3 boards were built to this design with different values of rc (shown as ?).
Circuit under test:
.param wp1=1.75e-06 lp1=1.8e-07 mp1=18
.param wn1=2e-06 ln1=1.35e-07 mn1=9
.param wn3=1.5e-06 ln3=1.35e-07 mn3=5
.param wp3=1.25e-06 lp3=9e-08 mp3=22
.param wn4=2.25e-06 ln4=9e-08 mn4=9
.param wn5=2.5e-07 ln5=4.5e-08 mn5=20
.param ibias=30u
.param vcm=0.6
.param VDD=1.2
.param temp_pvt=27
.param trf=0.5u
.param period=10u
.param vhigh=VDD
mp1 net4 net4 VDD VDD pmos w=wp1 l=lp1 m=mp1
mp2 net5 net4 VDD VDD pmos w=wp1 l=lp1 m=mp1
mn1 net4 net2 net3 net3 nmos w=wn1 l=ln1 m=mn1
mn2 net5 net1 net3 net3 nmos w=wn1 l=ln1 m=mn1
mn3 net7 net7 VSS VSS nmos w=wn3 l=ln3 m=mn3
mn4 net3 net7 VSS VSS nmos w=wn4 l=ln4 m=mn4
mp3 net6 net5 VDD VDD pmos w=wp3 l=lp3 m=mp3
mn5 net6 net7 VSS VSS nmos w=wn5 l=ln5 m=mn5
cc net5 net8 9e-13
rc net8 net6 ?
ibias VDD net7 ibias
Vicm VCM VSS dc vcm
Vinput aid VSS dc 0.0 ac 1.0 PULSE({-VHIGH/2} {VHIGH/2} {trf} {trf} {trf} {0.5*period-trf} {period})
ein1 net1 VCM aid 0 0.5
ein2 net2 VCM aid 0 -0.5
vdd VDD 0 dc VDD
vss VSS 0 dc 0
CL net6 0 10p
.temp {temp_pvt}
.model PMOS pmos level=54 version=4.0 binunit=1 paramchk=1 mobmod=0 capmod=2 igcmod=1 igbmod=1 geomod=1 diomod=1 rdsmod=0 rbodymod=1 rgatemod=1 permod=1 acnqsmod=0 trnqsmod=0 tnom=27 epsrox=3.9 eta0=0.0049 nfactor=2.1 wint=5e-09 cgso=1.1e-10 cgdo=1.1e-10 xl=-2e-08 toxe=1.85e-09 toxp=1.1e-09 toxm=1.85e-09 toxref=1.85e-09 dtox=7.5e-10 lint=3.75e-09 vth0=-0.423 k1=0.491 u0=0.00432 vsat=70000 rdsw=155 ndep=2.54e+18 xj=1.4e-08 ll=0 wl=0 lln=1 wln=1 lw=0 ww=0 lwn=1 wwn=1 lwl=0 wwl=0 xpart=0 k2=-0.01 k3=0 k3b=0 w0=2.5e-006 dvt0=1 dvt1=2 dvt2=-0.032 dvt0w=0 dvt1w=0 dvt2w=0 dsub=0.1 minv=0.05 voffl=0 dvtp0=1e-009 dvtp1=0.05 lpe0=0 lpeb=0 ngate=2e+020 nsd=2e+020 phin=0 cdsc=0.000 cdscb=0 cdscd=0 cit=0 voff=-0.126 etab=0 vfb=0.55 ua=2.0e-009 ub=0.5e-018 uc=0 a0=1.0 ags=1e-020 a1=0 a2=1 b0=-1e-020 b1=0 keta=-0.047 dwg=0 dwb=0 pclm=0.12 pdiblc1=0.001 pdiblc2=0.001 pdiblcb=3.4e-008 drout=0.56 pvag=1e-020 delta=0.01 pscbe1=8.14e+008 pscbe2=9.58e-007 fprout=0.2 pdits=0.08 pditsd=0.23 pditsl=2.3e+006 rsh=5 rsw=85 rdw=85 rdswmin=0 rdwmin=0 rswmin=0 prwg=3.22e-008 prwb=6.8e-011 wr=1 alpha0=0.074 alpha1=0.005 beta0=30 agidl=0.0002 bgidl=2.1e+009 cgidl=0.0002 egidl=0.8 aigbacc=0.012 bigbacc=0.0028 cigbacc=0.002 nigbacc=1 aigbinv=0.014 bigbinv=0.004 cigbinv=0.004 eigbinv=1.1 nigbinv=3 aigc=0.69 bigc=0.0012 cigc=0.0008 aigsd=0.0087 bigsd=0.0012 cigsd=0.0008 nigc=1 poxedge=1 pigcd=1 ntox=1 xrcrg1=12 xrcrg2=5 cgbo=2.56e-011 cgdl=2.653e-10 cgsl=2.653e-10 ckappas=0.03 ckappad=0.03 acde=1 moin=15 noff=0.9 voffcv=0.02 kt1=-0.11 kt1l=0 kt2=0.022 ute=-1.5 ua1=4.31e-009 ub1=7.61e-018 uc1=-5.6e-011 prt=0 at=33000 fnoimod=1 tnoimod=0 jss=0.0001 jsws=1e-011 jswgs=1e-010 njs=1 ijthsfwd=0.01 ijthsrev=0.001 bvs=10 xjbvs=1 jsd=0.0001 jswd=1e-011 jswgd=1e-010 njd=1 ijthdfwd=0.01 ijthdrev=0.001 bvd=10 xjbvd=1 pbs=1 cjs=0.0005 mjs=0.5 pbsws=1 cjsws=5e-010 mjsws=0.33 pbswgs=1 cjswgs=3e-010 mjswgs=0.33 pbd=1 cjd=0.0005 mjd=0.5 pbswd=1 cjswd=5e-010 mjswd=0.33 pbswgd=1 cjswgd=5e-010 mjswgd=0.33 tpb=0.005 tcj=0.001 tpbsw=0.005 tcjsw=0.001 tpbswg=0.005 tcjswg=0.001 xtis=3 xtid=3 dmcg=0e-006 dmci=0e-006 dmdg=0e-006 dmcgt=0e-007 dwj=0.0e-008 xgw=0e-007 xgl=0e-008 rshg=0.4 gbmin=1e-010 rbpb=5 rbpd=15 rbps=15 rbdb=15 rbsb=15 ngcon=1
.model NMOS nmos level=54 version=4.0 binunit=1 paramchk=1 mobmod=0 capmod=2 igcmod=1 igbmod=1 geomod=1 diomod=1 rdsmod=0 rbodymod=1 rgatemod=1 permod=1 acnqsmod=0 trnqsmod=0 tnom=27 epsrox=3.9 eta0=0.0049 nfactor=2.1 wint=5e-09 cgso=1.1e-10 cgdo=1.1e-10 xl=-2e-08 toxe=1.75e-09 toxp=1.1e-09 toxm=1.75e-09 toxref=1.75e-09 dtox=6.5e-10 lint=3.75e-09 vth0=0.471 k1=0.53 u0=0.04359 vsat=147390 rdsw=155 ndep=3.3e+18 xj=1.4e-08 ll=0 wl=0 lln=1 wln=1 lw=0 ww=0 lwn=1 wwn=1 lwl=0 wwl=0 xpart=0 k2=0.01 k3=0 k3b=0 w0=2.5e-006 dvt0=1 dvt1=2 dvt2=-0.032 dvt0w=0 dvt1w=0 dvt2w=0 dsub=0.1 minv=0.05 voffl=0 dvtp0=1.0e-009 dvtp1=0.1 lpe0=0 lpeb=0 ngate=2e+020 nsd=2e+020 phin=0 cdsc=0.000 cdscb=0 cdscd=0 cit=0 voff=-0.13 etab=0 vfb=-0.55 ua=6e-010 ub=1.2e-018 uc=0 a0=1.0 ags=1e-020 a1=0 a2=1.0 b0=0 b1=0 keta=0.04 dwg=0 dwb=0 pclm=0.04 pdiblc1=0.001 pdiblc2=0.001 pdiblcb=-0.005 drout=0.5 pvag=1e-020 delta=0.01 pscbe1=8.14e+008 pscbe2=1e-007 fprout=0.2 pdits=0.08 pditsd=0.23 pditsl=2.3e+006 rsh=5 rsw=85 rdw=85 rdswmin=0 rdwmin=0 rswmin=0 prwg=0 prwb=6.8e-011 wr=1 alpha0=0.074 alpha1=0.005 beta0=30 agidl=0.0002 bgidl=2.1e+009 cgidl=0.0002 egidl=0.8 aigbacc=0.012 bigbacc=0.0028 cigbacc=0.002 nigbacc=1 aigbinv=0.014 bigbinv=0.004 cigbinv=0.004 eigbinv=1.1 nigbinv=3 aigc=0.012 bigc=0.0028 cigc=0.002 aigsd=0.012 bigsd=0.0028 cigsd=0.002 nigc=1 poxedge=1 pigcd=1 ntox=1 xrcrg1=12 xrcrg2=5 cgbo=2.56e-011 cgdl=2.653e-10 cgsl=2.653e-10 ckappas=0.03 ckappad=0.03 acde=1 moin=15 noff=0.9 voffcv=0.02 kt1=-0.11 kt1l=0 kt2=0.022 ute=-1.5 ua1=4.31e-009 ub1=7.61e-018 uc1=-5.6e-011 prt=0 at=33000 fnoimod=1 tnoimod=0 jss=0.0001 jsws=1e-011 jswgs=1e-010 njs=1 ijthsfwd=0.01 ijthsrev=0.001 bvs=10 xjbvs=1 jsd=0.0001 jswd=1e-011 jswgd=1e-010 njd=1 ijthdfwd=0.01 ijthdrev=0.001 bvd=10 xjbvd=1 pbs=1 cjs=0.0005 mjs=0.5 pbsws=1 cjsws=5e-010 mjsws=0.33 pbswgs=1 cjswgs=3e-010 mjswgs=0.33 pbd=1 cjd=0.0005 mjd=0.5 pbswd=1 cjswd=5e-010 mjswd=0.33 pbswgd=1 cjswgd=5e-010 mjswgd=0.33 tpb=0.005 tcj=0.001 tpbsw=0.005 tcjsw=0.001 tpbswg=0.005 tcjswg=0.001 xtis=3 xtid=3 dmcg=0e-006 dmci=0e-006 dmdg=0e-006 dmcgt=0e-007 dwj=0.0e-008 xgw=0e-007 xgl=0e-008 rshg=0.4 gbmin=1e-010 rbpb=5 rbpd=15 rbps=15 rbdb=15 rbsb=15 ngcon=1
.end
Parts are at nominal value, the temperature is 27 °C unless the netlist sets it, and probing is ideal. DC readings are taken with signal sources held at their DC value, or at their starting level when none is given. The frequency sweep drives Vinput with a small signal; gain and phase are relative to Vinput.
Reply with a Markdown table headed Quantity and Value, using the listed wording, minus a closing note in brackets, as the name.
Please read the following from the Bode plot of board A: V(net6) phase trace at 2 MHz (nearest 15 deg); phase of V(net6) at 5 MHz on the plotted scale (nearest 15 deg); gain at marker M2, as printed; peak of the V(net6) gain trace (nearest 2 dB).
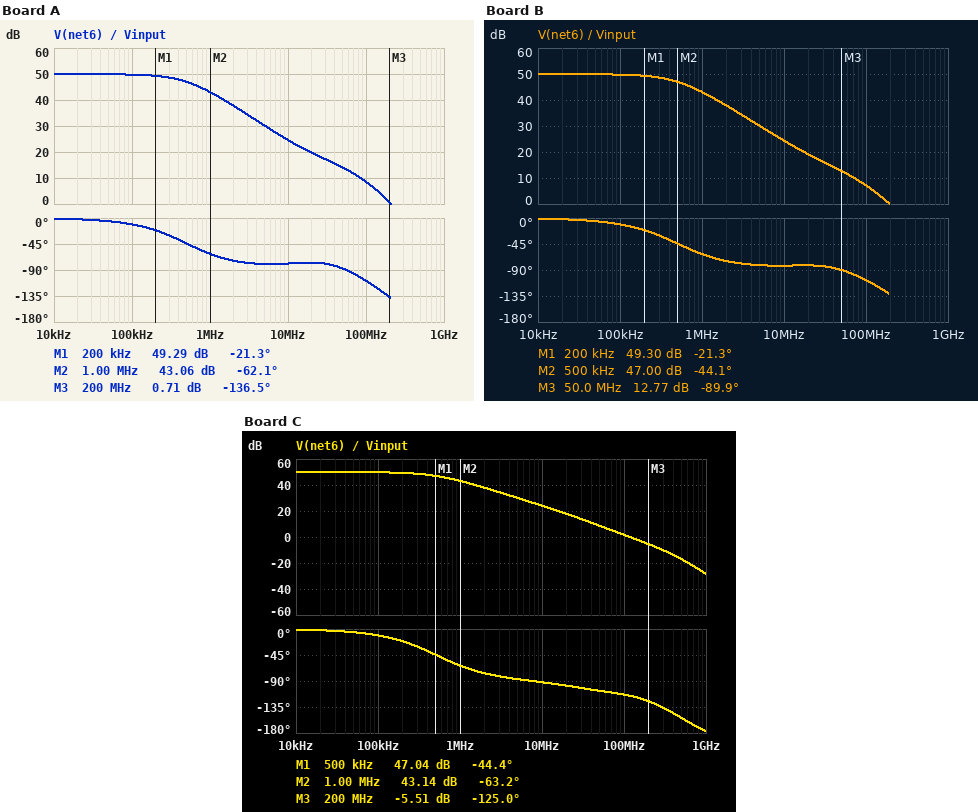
| Quantity | Value |
|---|---|
| V(net6) phase trace at 2 MHz | -75 deg |
| phase of V(net6) at 5 MHz on the plotted scale | -75 deg |
| gain at marker M2, as printed | 43.06 dB |
| peak of the V(net6) gain trace | 50 dB |
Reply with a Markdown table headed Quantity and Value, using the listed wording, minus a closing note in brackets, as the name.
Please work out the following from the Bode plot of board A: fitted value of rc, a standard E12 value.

| Quantity | Value |
|---|---|
| fitted value of rc, a standard E12 value | 8.2 kΩ |
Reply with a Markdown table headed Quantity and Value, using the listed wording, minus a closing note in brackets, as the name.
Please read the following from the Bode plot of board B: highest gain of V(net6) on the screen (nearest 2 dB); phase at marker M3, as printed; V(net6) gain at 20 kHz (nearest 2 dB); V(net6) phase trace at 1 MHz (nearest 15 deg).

| Quantity | Value |
|---|---|
| highest gain of V(net6) on the screen | 50 dB |
| phase at marker M3, as printed | -89.9 deg |
| V(net6) gain at 20 kHz | 50 dB |
| V(net6) phase trace at 1 MHz | -60 deg |
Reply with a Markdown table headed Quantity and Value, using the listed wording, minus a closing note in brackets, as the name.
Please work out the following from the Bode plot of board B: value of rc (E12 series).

| Quantity | Value |
|---|---|
| value of rc | 6.8 kΩ |
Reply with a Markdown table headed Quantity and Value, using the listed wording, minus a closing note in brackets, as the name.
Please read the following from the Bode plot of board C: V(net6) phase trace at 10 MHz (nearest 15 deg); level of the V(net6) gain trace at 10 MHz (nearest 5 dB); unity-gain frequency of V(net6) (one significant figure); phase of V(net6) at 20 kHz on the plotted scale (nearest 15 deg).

| Quantity | Value |
|---|---|
| V(net6) phase trace at 10 MHz | -90 deg |
| level of the V(net6) gain trace at 10 MHz | 25 dB |
| unity-gain frequency of V(net6) | 100 MHz |
| phase of V(net6) at 20 kHz on the plotted scale | 0 deg |
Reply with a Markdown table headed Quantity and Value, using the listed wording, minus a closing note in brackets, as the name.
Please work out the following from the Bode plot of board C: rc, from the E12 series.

| Quantity | Value |
|---|---|
| rc, from the E12 series | 3.3 kΩ |
